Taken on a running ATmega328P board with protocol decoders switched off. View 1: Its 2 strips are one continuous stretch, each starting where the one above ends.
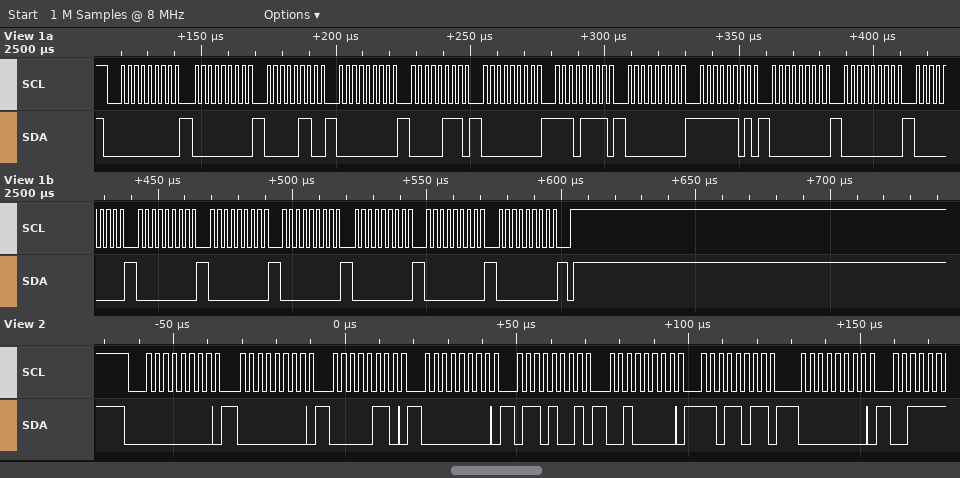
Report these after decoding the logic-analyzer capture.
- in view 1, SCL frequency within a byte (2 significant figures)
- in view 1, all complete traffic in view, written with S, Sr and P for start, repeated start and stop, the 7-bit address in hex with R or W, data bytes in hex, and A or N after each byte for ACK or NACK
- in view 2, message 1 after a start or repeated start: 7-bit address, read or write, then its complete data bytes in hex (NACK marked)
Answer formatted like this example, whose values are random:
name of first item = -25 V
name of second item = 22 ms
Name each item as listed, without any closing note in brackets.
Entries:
in view 1, SCL frequency within a byte = 400 kHz
in view 1, all complete traffic in view, written with S, Sr and P for start, repeated start and stop, the 7-bit address in hex with R or W, data bytes in hex, and A or N after each byte for ACK or NACK = S 00W A 00 A 06 A 00 A 07 A 00 A EF A 00 A FD A 00 A 00 A 00 A 00 A 00 A 00 A 00 A 00 A 00 A P
in view 2, message 1 after a start or repeated start: 7-bit address, read or write, then its complete data bytes in hex = 0x00 write: 00 06 00 69 20 DB 00
